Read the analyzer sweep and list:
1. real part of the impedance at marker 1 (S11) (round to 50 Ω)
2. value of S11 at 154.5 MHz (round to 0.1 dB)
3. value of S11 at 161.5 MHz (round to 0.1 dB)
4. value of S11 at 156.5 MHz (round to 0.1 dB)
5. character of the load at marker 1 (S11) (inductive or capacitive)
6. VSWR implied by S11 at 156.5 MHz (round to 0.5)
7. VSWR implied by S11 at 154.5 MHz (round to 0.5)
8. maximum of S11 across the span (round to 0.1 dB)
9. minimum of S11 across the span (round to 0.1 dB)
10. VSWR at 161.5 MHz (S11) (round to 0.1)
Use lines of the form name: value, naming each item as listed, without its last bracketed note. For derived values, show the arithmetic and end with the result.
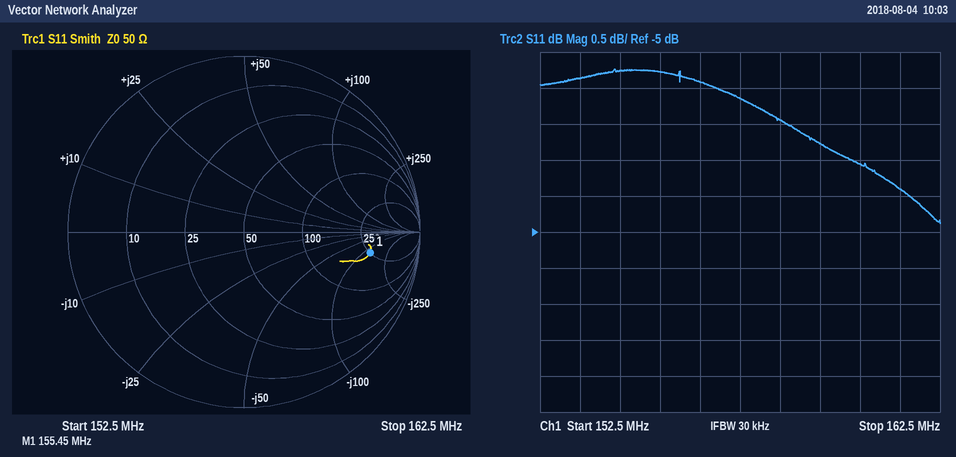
real part of the impedance at marker 1 (S11): 250 Ω
value of S11 at 154.5 MHz: -2.8 dB
value of S11 at 161.5 MHz: -4.4 dB
value of S11 at 156.5 MHz: -2.9 dB
character of the load at marker 1 (S11): capacitive
VSWR implied by S11 at 156.5 MHz: |Γ| = 10^(-2.9/20) = 0.7161; VSWR = (1 + 0.7161)/(1 − 0.7161) ≈ 6.0
VSWR implied by S11 at 154.5 MHz: |Γ| = 10^(-2.8/20) = 0.7244; VSWR = (1 + 0.7244)/(1 − 0.7244) ≈ 6.26, so 6.5 to the nearest 0.5
maximum of S11 across the span: -2.7 dB
minimum of S11 across the span: -4.9 dB
VSWR at 161.5 MHz (S11): |Γ| = 10^(-4.4/20) = 0.6026; VSWR = (1 + 0.6026)/(1 − 0.6026) ≈ 4.0
